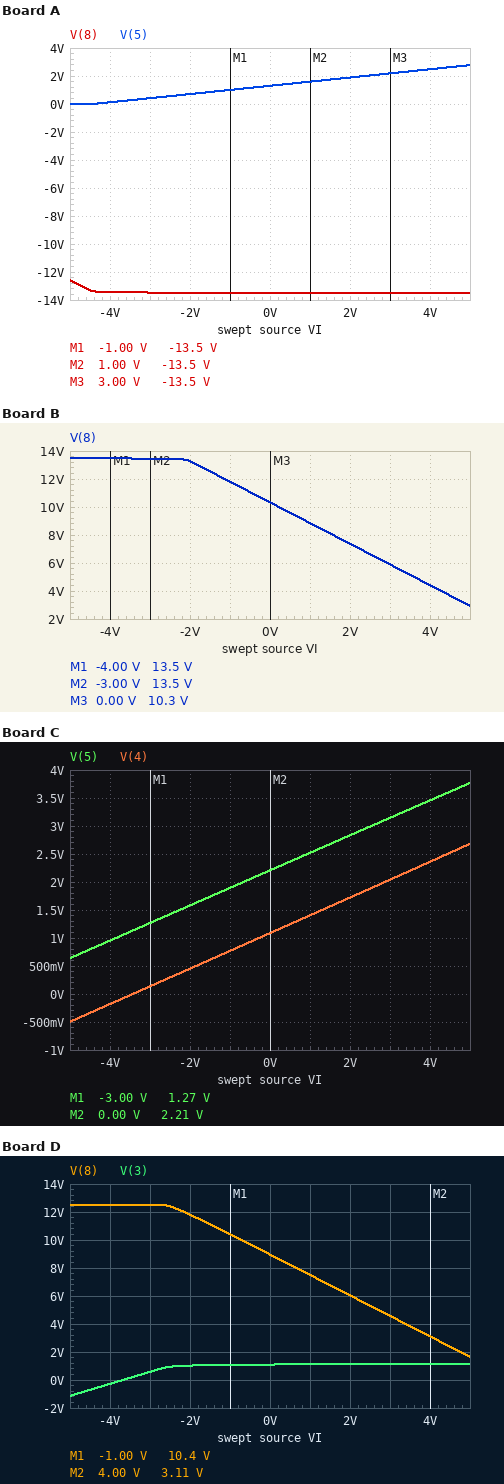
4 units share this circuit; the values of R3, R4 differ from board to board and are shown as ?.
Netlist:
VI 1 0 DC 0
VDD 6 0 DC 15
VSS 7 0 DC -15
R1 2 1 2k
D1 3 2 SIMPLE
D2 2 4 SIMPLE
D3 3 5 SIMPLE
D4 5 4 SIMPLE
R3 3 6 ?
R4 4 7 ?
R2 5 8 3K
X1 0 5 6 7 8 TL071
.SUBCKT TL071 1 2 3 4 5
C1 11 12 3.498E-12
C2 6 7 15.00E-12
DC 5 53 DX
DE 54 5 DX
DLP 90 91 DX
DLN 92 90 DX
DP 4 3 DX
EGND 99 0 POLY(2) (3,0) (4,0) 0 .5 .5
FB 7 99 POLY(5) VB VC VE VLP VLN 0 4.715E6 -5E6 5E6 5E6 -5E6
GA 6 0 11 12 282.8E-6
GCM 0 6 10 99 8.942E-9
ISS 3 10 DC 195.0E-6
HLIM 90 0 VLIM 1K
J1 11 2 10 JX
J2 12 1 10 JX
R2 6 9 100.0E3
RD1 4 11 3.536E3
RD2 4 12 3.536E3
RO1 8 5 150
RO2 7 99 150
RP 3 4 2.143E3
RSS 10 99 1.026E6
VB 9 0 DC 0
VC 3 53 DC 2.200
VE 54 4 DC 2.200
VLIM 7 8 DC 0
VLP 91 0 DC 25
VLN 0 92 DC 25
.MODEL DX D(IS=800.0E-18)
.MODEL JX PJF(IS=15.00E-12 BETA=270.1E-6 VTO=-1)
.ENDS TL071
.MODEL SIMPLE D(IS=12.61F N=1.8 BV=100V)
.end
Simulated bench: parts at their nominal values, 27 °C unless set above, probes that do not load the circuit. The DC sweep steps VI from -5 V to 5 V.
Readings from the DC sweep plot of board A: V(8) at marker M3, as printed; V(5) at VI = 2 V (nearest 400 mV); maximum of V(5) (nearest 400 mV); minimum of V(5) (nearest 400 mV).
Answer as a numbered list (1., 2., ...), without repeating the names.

1. -13.5 V
2. 2.0 V
3. 2.8 V
4. 0 V
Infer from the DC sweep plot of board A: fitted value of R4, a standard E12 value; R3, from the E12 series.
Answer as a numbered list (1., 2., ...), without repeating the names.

1. 5.6 kΩ
2. 1.5 kΩ
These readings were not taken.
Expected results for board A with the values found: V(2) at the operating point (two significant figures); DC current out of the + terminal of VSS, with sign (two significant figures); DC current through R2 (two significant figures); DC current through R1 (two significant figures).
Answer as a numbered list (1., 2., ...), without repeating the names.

1. 1.3 V
2. -17 mA
3. 4.9 mA
4. 670 µA
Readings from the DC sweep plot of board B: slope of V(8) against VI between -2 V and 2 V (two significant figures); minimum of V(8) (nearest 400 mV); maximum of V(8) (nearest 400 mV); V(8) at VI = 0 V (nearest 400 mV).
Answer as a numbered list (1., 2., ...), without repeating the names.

1. -1.5 V/V
2. 2.8 V
3. 13.6 V
4. 10.4 V
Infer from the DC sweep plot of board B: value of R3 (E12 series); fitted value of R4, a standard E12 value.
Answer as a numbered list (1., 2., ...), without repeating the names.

1. 3.3 kΩ
2. 1.8 kΩ
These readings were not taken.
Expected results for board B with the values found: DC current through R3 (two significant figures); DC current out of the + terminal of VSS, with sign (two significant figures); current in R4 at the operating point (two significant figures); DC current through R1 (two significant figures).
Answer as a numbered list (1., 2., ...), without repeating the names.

1. 4.2 mA
2. -22 mA
3. 7.6 mA
4. 14 µA
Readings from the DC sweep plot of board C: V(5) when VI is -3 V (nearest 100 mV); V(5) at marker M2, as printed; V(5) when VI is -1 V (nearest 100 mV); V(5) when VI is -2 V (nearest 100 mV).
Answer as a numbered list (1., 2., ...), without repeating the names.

1. 1.3 V
2. 2.21 V
3. 1.9 V
4. 1.6 V
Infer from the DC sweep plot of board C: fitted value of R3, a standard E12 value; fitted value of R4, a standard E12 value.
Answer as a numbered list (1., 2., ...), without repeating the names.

1. 1.5 kΩ
2. 12 kΩ
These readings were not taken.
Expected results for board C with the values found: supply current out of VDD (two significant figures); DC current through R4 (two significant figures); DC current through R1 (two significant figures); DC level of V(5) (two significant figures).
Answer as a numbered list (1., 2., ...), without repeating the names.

1. 22 mA
2. 1.3 mA
3. 1.1 mA
4. 2.2 V
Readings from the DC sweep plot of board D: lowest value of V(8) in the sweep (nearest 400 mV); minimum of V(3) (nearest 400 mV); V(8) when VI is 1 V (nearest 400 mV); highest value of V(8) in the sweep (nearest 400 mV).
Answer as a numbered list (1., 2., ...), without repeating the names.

1. 1.6 V
2. -1.2 V
3. 7.6 V
4. 12.4 V
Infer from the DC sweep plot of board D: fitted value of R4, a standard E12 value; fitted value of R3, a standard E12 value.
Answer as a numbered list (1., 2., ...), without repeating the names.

1. 3.3 kΩ
2. 12 kΩ
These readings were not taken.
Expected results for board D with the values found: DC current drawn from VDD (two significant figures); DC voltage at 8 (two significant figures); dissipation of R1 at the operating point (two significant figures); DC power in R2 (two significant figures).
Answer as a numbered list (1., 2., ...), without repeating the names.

1. 15 mA
2. 9.0 V
3. 1.7 µW
4. 27 mW
